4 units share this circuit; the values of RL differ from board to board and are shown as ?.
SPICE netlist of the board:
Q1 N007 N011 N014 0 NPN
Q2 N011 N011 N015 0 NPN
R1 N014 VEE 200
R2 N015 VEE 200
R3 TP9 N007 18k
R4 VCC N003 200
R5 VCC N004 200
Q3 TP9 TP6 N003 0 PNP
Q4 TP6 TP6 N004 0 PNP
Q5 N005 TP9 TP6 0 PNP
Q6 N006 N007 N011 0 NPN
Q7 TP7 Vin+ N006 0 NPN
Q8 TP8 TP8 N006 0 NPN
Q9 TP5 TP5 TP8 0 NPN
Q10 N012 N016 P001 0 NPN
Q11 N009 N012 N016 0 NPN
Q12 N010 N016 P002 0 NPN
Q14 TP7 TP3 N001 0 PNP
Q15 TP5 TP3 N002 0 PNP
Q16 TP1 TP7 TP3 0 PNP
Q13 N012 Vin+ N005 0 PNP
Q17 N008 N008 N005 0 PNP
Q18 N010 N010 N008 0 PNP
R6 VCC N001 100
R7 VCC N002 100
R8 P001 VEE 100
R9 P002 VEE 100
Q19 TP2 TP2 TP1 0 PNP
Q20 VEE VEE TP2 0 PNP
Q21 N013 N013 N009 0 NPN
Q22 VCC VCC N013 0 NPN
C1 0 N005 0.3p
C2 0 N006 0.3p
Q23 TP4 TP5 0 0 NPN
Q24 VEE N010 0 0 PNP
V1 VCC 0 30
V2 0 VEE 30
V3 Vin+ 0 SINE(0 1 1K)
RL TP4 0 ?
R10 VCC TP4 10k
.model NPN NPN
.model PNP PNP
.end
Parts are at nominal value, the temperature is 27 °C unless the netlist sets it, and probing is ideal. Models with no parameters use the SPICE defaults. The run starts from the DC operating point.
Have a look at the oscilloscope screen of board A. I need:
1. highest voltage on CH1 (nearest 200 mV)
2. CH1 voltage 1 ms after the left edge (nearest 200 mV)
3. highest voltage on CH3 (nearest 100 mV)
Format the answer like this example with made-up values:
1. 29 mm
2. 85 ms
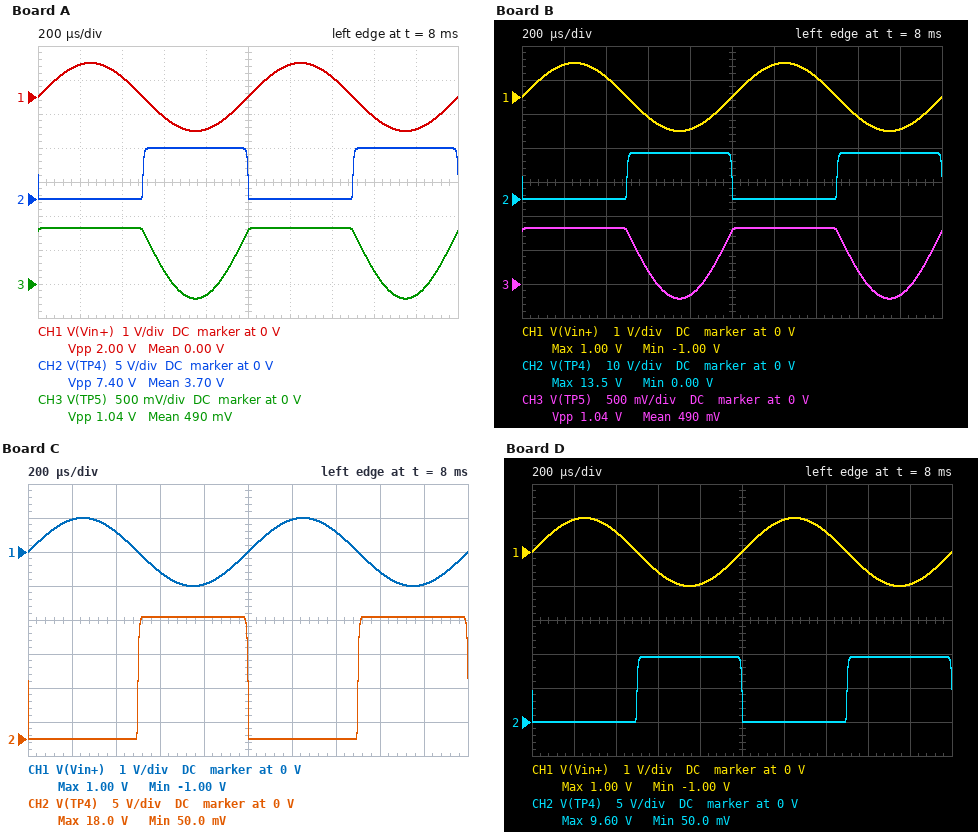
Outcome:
1. 1.0 V
2. 0 V
3. 800 mV
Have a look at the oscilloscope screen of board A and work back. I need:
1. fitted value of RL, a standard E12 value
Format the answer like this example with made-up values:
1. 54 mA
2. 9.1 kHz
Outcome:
1. 3.3 kΩ
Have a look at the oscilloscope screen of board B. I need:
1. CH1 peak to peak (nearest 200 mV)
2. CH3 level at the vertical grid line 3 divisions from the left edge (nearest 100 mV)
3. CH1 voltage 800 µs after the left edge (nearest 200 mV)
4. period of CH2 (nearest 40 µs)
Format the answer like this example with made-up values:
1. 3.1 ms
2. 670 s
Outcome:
1. 2.0 V
2. 200 mV
3. -1.0 V
4. 1.00 ms
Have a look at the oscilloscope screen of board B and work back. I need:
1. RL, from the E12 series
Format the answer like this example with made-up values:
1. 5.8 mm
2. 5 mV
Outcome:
1. 8.2 kΩ
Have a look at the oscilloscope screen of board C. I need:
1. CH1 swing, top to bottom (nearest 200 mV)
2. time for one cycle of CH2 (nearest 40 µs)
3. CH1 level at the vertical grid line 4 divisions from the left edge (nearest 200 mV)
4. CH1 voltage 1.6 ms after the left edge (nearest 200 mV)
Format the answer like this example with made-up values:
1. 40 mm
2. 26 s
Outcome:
1. 2.0 V
2. 1.00 ms
3. -1.0 V
4. -600 mV
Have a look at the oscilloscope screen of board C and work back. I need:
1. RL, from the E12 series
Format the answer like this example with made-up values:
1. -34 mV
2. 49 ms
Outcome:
1. 15 kΩ
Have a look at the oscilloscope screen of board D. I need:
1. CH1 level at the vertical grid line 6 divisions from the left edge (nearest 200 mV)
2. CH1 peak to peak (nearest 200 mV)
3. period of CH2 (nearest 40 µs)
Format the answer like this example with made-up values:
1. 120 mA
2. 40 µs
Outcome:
1. 1.0 V
2. 2.0 V
3. 1.00 ms
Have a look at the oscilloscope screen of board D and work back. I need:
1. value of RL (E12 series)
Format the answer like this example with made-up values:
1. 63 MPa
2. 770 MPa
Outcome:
1. 4.7 kΩ
